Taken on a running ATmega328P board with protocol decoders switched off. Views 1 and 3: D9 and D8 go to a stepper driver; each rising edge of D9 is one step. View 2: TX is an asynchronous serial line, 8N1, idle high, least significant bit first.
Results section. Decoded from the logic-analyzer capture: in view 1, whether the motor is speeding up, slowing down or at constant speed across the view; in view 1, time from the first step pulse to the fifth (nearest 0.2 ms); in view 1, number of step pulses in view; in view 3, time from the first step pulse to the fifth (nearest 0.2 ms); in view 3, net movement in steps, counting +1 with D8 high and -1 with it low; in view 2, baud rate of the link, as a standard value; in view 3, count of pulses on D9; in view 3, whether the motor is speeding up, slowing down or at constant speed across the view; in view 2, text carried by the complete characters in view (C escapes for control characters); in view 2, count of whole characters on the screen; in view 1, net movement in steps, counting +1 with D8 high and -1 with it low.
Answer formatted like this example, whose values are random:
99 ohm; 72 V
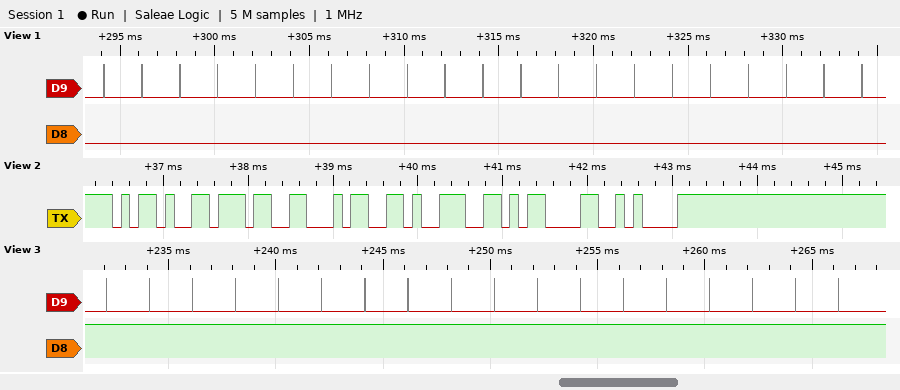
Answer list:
constant speed; 8.0 ms; 21; 8.0 ms; +18; 9600 baud; 18; constant speed; "-749\r\n"; 6; -21
